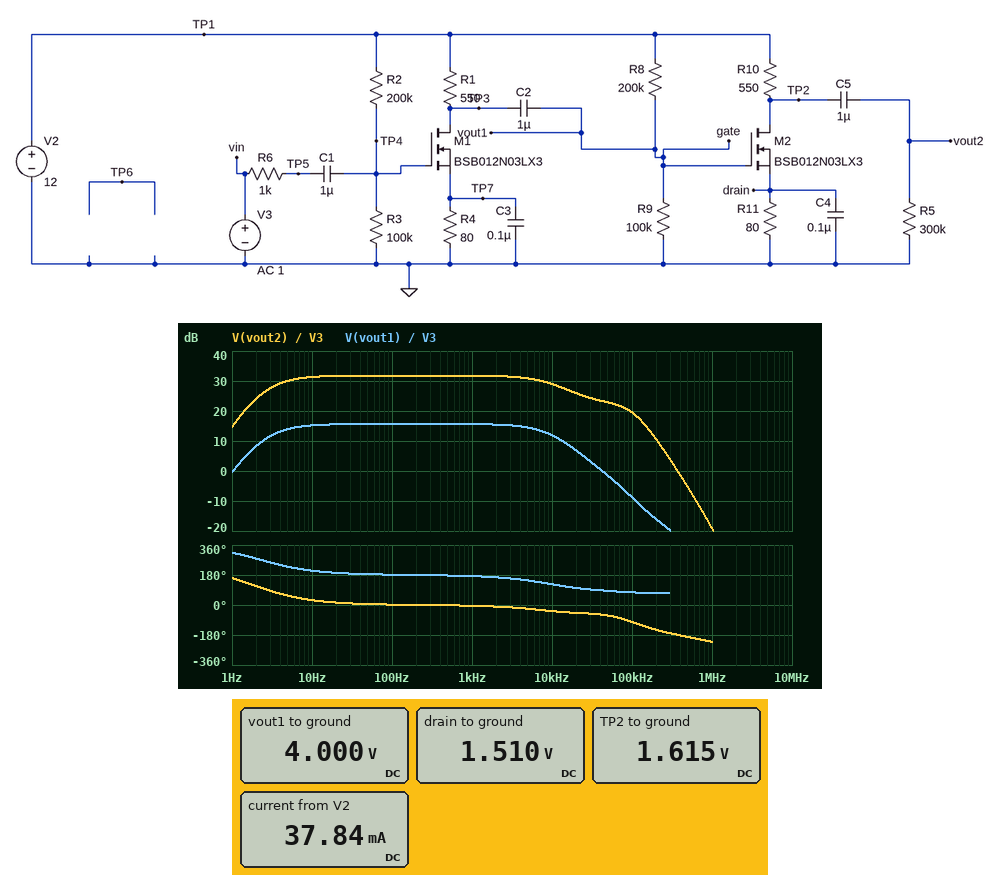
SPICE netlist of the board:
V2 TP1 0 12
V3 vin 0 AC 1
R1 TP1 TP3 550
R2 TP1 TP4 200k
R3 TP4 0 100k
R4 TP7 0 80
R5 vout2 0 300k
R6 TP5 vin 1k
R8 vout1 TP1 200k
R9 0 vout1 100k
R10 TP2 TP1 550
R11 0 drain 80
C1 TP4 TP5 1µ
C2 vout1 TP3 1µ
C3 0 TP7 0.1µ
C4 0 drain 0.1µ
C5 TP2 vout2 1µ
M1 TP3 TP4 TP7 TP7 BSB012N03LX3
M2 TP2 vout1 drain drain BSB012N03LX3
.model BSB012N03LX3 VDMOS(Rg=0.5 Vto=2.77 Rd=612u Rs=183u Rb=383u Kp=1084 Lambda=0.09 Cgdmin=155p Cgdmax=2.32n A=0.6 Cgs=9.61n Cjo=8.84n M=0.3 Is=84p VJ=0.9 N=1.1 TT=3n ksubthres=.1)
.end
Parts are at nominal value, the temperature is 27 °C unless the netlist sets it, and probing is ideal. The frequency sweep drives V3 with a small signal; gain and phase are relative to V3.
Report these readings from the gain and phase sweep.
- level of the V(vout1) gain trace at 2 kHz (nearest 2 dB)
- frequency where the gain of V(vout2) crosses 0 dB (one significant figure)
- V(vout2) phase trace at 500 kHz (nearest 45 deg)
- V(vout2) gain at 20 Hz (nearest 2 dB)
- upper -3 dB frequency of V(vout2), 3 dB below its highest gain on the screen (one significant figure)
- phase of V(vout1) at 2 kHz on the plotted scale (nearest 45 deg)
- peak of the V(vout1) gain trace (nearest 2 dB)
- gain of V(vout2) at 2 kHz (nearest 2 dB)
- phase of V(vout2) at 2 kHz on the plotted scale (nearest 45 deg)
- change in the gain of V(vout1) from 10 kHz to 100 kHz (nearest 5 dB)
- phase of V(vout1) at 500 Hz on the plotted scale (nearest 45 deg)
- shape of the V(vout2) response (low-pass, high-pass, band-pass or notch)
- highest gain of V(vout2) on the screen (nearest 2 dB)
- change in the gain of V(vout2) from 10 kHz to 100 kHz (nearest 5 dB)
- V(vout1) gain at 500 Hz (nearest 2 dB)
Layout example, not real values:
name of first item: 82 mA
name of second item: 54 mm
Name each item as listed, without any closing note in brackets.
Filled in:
level of the V(vout1) gain trace at 2 kHz: 16 dB
frequency where the gain of V(vout2) crosses 0 dB: 400 kHz
V(vout2) phase trace at 500 kHz: -180 deg
V(vout2) gain at 20 Hz: 32 dB
upper -3 dB frequency of V(vout2), 3 dB below its highest gain on the screen: 10 kHz
phase of V(vout1) at 2 kHz on the plotted scale: 180 deg
peak of the V(vout1) gain trace: 16 dB
gain of V(vout2) at 2 kHz: 32 dB
phase of V(vout2) at 2 kHz on the plotted scale: 0 deg
change in the gain of V(vout1) from 10 kHz to 100 kHz: -20 dB
phase of V(vout1) at 500 Hz on the plotted scale: 180 deg
shape of the V(vout2) response: band-pass
highest gain of V(vout2) on the screen: 32 dB
change in the gain of V(vout2) from 10 kHz to 100 kHz: -10 dB
V(vout1) gain at 500 Hz: 16 dB
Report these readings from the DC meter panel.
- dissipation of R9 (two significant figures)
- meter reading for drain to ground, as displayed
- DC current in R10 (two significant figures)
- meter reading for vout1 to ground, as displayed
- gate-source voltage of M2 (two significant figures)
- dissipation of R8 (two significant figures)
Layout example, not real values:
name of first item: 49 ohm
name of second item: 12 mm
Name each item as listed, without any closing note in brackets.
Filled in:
dissipation of R9: 160 µW
meter reading for drain to ground, as displayed: 1.510 V
DC current in R10: 19 mA
meter reading for vout1 to ground, as displayed: 4.000 V
gate-source voltage of M2: 2.5 V
dissipation of R8: 320 µW
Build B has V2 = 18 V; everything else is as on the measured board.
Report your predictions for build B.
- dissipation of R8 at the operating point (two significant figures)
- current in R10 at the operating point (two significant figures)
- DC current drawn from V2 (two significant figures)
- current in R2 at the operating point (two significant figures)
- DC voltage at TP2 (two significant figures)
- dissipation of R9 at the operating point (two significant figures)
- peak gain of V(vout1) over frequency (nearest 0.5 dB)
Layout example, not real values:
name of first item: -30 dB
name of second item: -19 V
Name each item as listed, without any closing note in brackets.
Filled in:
dissipation of R8 at the operating point: 720 µW
current in R10 at the operating point: 29 mA
DC current drawn from V2: 57 mA
current in R2 at the operating point: 60 µA
DC voltage at TP2: 2.3 V
dissipation of R9 at the operating point: 360 µW
peak gain of V(vout1) over frequency: -28.0 dB
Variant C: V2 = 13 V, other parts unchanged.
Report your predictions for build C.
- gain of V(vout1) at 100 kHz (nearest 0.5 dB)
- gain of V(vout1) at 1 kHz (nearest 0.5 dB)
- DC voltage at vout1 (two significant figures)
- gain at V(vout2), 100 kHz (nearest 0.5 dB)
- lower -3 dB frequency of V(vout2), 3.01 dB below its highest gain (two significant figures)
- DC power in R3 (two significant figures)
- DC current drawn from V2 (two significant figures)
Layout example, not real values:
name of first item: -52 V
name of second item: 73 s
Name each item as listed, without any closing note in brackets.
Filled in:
gain of V(vout1) at 100 kHz: -37.5 dB
gain of V(vout1) at 1 kHz: -44.0 dB
DC voltage at vout1: 4.3 V
gain at V(vout2), 100 kHz: -57.5 dB
lower -3 dB frequency of V(vout2), 3.01 dB below its highest gain: 13 kHz
DC power in R3: 190 µW
DC current drawn from V2: 41 mA
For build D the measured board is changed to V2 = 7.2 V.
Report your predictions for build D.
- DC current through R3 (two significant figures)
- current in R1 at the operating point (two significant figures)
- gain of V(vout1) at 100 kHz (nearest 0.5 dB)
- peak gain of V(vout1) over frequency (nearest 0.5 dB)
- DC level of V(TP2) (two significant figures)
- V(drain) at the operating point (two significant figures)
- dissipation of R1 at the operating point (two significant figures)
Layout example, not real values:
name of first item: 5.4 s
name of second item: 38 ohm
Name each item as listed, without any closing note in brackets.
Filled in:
DC current through R3: 24 µA
current in R1 at the operating point: 1.0 mA
gain of V(vout1) at 100 kHz: -11.0 dB
peak gain of V(vout1) over frequency: 13.0 dB
DC level of V(TP2): 6.6 V
V(drain) at the operating point: 82 mV
dissipation of R1 at the operating point: 570 µW
